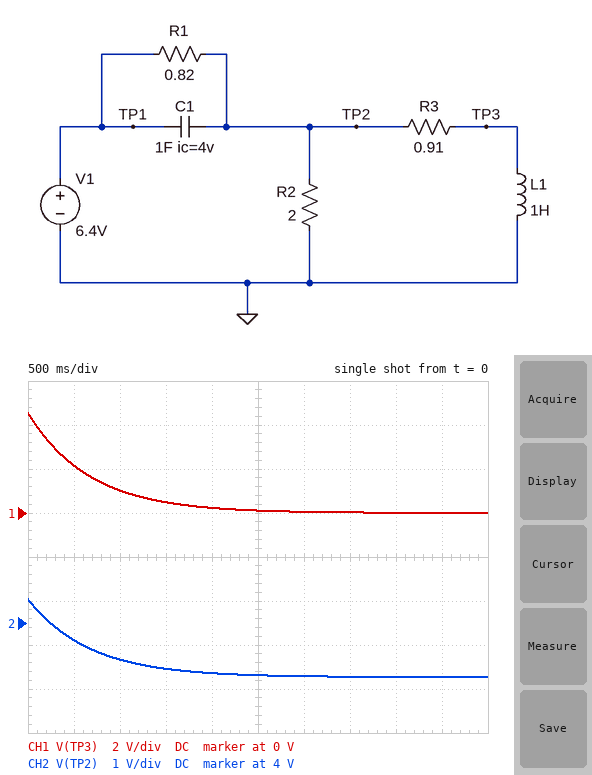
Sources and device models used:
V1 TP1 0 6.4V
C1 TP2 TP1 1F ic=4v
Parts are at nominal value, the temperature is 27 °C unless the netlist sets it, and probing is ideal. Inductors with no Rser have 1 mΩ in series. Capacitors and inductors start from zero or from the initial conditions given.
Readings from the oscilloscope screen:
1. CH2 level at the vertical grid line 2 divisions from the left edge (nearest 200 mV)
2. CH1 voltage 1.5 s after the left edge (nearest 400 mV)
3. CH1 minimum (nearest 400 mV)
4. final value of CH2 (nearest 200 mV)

3.2 V
400 mV
0 V
2.8 V
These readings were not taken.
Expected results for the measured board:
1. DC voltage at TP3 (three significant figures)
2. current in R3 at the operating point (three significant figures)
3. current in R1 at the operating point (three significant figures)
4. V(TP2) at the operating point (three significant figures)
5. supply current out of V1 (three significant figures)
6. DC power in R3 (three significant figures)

3.04 mV
3.04 A
4.43 A
2.77 V
4.43 A
8.42 W
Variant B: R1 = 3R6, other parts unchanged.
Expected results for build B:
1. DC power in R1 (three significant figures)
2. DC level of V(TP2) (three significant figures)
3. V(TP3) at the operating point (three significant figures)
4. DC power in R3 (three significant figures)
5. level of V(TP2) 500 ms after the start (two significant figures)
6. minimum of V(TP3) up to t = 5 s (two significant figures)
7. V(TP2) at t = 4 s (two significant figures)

8.26 W
948 mV
1.04 mV
985 mW
1.4 V
1.1 mV
950 mV
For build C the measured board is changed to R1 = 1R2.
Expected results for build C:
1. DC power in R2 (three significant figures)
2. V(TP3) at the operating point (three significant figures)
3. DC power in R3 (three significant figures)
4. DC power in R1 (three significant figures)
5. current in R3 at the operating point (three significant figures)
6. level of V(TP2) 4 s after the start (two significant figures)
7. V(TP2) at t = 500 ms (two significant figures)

2.41 W
2.41 mV
5.28 W
14.7 W
2.41 A
2.2 V
3.0 V
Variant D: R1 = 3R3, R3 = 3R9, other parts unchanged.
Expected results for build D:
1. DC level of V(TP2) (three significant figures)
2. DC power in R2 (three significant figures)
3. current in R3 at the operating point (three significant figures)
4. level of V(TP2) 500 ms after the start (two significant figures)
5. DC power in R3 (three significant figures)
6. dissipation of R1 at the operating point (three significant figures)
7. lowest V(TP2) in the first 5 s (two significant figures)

1.83 V
1.68 W
469 mA
1.9 V
859 mW
6.33 W
1.8 V
